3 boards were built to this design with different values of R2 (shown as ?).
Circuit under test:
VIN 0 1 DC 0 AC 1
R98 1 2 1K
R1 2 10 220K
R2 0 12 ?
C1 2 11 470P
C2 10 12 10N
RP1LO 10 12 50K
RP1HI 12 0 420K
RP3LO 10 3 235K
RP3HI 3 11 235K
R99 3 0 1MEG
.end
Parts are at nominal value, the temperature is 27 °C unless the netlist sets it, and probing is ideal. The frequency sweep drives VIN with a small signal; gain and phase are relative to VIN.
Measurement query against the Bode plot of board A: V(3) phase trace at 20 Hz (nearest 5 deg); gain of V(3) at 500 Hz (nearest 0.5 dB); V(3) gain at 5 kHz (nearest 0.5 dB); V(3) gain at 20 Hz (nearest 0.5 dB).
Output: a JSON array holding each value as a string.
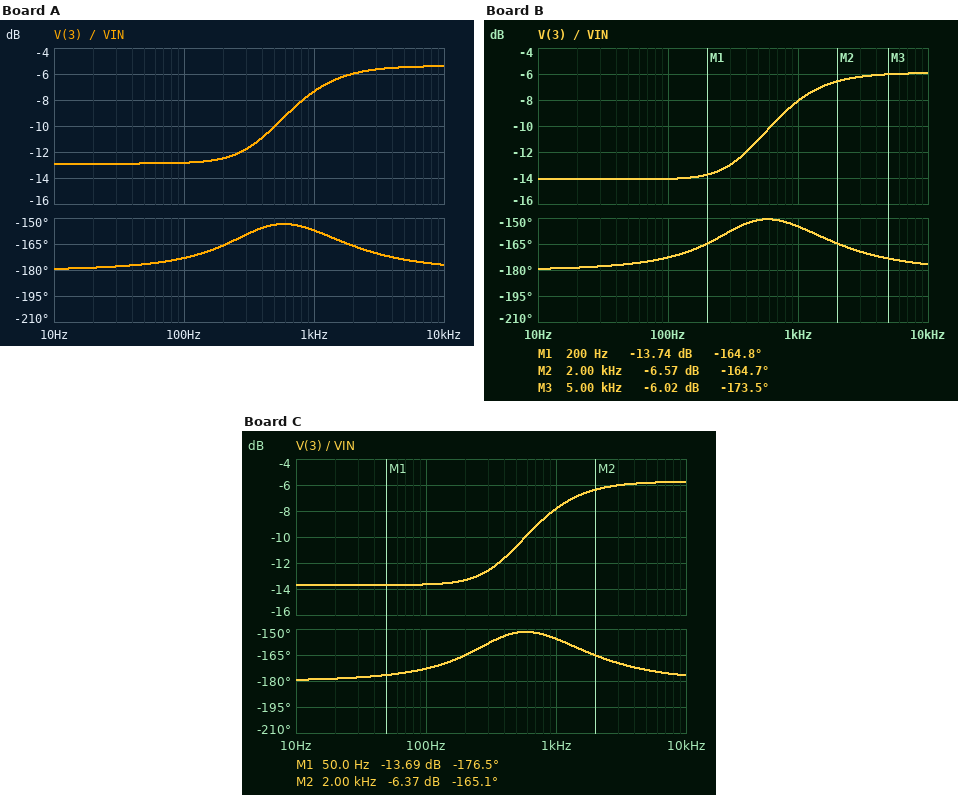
["-180 deg", "-10.0 dB", "-5.5 dB", "-13.0 dB"]
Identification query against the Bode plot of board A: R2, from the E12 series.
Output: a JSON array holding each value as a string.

["47 kΩ"]
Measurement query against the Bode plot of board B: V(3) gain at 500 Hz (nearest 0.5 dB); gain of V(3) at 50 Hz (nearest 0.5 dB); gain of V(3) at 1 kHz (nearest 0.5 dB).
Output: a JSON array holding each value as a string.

["-11.0 dB", "-14.0 dB", "-8.0 dB"]
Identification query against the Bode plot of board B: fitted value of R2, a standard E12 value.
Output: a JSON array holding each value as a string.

["27 kΩ"]
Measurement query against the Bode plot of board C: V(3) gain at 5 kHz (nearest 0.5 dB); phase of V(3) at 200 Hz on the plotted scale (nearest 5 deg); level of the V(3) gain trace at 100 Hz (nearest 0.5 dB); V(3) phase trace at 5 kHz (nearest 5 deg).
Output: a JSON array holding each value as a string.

["-6.0 dB", "-165 deg", "-13.5 dB", "-175 deg"]
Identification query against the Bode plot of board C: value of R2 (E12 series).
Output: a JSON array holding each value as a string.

["33 kΩ"]
